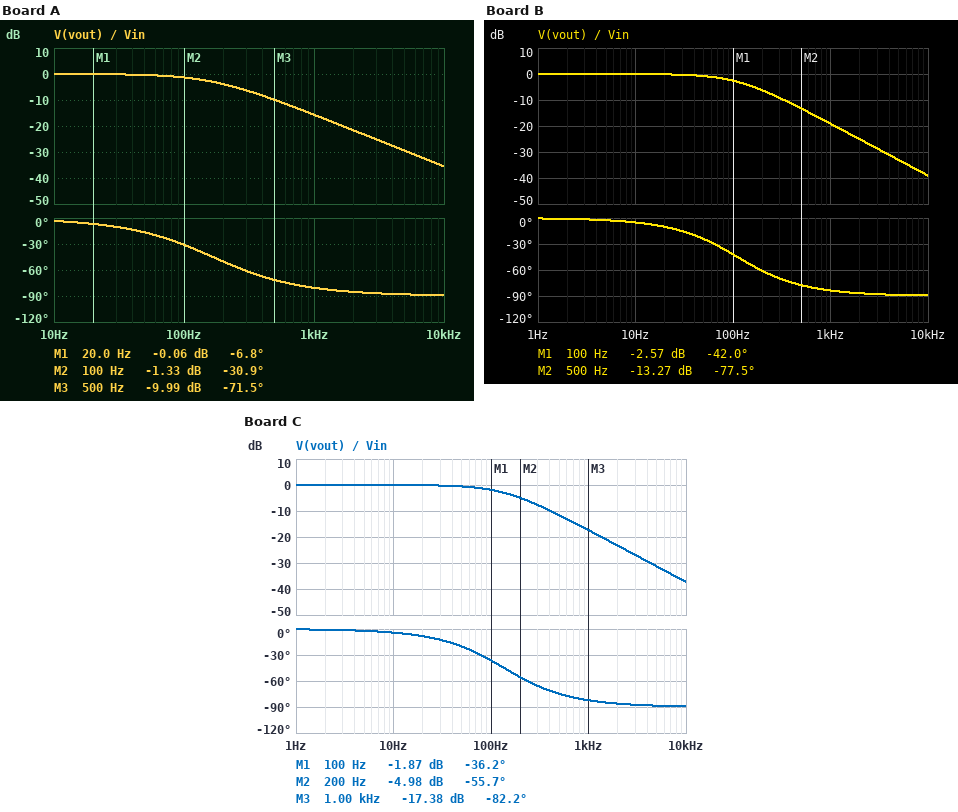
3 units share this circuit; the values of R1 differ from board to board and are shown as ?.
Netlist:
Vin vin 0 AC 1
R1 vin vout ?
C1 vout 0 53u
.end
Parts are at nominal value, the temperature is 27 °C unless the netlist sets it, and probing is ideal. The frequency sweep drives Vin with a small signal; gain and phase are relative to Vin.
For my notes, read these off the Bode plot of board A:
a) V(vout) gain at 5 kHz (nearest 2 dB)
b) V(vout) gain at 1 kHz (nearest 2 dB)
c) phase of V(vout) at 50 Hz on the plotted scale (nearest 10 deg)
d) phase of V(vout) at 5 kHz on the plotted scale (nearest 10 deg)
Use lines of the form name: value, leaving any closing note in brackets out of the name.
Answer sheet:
V(vout) gain at 5 kHz: -30 dB
V(vout) gain at 1 kHz: -16 dB
phase of V(vout) at 50 Hz on the plotted scale: -20 deg
phase of V(vout) at 5 kHz on the plotted scale: -90 deg
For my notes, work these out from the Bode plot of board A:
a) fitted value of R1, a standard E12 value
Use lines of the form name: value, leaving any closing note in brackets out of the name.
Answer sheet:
fitted value of R1, a standard E12 value: 18 Ω
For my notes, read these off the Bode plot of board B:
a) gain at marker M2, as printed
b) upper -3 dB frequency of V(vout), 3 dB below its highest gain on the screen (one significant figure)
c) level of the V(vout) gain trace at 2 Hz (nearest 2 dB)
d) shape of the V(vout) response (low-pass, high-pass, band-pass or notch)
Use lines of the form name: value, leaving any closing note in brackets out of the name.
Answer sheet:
gain at marker M2, as printed: -13.27 dB
upper -3 dB frequency of V(vout), 3 dB below its highest gain on the screen: 100 Hz
level of the V(vout) gain trace at 2 Hz: 0 dB
shape of the V(vout) response: low-pass
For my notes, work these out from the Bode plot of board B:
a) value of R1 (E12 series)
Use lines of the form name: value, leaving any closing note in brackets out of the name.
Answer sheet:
value of R1: 27 Ω
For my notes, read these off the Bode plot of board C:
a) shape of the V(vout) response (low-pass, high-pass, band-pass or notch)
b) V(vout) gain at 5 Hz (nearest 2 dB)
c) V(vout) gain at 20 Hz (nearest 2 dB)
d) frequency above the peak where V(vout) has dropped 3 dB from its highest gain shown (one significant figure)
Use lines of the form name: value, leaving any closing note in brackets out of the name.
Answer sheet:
shape of the V(vout) response: low-pass
V(vout) gain at 5 Hz: 0 dB
V(vout) gain at 20 Hz: 0 dB
frequency above the peak where V(vout) has dropped 3 dB from its highest gain shown: 100 Hz
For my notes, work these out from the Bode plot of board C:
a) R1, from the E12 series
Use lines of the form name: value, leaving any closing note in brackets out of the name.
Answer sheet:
R1, from the E12 series: 22 Ω
